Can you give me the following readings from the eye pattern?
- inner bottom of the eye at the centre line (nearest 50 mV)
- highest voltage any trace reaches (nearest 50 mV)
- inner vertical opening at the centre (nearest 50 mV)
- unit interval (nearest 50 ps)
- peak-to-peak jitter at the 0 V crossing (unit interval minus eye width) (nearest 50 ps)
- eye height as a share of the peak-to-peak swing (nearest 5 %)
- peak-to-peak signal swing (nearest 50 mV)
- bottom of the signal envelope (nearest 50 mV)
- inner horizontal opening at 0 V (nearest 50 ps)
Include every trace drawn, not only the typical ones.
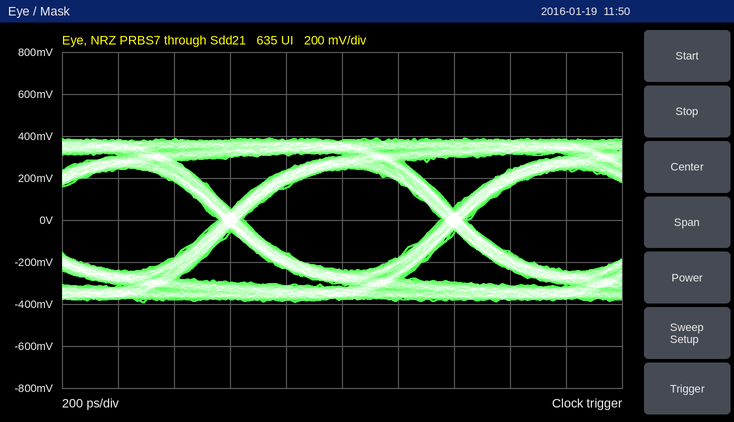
-250 mV
400 mV
500 mV
800 ps
100 ps
60 %
800 mV
-400 mV
700 ps
